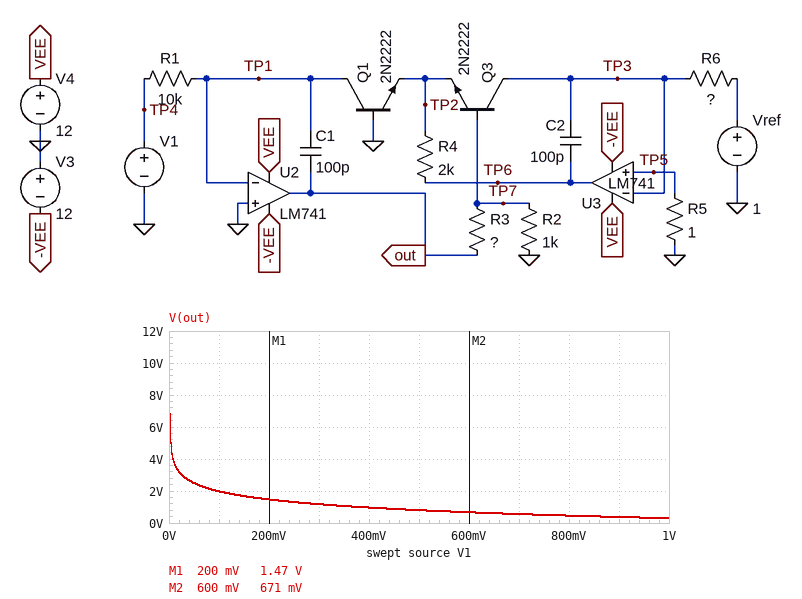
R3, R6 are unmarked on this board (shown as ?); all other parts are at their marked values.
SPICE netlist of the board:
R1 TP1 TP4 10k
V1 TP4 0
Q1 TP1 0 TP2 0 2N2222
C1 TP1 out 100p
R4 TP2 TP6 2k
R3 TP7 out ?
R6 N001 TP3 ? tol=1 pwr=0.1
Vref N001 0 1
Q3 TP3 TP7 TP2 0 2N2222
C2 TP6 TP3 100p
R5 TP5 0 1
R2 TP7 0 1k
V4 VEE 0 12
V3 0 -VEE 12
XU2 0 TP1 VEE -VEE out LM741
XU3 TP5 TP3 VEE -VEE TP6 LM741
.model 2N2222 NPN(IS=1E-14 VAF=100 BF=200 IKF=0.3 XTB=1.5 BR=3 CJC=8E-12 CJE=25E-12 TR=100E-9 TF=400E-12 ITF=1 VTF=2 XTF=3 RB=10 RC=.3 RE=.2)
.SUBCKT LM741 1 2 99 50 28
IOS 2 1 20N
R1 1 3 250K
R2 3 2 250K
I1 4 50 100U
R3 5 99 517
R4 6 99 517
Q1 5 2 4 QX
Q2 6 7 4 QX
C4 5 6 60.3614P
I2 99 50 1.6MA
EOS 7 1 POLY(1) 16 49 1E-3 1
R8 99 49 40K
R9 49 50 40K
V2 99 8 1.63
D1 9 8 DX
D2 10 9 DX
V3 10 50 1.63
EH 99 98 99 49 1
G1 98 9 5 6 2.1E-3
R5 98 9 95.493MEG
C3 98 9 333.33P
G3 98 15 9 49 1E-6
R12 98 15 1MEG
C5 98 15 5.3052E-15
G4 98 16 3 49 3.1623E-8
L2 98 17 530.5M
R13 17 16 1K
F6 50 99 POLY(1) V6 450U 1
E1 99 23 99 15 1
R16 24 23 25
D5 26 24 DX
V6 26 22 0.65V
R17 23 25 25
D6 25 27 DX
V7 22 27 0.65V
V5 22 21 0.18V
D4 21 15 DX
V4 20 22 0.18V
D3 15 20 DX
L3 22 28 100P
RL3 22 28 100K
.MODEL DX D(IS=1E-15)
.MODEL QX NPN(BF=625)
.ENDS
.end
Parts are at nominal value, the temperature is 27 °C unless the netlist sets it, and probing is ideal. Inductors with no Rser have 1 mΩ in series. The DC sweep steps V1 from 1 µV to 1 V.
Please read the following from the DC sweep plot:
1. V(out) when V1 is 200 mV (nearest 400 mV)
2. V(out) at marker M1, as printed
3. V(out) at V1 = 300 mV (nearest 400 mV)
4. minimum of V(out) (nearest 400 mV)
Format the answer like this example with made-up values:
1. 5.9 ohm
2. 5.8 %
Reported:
1. 1.6 V
2. 1.47 V
3. 1.2 V
4. 400 mV
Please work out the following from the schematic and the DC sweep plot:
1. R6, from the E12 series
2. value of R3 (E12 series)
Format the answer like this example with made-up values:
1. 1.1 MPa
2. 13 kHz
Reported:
1. 6.8 kΩ
2. 27 kΩ
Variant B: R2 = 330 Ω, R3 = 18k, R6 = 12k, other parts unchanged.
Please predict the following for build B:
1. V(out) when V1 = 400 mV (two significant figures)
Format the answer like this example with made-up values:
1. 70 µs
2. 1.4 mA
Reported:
1. 1.1 V
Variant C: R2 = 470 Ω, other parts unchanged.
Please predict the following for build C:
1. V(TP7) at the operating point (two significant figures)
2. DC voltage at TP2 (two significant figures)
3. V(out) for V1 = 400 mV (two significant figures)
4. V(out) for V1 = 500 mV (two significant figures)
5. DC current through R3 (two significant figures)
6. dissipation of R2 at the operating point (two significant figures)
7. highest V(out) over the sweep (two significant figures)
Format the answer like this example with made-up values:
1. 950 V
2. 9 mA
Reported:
1. 190 mV
2. -420 mV
3. 2.0 V
4. 1.7 V
5. 400 µA
6. 74 µW
7. 11 V
